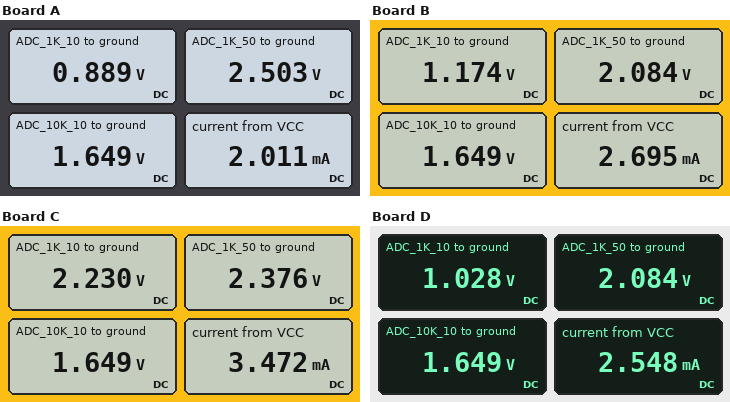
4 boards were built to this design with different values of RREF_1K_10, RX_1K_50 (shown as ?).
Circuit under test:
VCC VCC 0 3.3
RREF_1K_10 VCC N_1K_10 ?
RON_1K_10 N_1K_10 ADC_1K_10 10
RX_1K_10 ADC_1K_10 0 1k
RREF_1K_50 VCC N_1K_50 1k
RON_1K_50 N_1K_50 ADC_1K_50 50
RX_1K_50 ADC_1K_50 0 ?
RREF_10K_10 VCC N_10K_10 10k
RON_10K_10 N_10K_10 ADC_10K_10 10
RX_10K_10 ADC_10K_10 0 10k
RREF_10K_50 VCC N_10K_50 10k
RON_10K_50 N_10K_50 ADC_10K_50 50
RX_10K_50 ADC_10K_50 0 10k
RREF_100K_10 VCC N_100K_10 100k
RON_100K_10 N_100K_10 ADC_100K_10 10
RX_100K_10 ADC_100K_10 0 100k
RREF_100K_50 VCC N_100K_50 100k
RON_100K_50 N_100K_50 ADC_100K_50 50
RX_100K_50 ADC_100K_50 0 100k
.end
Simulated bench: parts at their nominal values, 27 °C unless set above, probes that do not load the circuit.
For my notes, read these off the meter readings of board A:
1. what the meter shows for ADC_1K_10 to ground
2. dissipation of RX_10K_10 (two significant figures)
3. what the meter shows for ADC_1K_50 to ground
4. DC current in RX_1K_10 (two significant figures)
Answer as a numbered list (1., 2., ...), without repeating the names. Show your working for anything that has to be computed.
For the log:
1. 0.889 V
2. (1.649 V)^2 / 10 kΩ = 270 µW
3. 2.503 V
4. (889 mV) / 1 kΩ = 890 µA
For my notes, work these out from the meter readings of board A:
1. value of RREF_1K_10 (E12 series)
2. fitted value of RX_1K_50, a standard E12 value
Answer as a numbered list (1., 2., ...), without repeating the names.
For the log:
1. 2.7 kΩ
2. 3.3 kΩ
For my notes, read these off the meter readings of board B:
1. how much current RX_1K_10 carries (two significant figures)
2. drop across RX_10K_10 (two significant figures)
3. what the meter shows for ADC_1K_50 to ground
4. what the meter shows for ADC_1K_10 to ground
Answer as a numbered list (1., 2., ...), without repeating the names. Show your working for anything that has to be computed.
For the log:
1. (1.174 V) / 1 kΩ = 1.2 mA
2. 1.649 V = 1.6 V
3. 2.084 V
4. 1.174 V
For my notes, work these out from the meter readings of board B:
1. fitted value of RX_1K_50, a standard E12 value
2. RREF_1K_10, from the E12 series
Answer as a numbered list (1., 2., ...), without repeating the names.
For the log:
1. 1.8 kΩ
2. 1.8 kΩ
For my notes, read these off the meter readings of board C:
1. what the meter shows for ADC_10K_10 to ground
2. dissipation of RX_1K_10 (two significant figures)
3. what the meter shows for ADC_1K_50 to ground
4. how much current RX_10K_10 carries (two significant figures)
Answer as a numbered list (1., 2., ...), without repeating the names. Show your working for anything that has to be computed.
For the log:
1. 1.649 V
2. (2.23 V)^2 / 1 kΩ = 5.0 mW
3. 2.376 V
4. (1.649 V) / 10 kΩ = 160 µA
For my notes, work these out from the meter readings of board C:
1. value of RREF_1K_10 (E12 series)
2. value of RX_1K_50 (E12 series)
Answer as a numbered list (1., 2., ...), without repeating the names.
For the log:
1. 470 Ω
2. 2.7 kΩ
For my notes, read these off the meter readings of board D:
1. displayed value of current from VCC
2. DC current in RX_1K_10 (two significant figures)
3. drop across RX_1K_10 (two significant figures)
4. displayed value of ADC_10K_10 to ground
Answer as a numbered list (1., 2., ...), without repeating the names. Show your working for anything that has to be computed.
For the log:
1. 2.548 mA
2. (1.028 V) / 1 kΩ = 1.0 mA
3. 1.028 V = 1.0 V
4. 1.649 V
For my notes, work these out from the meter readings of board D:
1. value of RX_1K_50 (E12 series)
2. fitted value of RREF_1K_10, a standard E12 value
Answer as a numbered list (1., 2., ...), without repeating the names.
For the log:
1. 1.8 kΩ
2. 2.2 kΩ
